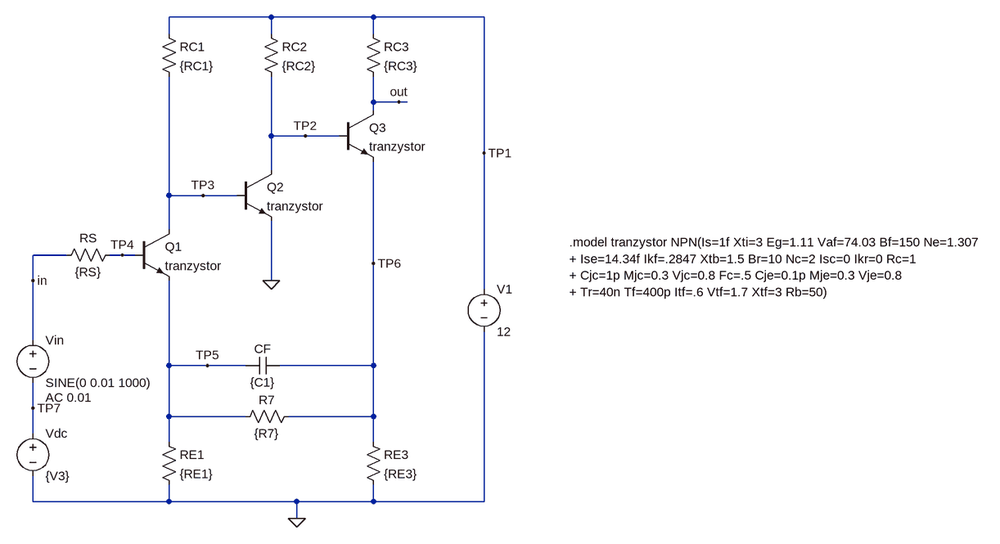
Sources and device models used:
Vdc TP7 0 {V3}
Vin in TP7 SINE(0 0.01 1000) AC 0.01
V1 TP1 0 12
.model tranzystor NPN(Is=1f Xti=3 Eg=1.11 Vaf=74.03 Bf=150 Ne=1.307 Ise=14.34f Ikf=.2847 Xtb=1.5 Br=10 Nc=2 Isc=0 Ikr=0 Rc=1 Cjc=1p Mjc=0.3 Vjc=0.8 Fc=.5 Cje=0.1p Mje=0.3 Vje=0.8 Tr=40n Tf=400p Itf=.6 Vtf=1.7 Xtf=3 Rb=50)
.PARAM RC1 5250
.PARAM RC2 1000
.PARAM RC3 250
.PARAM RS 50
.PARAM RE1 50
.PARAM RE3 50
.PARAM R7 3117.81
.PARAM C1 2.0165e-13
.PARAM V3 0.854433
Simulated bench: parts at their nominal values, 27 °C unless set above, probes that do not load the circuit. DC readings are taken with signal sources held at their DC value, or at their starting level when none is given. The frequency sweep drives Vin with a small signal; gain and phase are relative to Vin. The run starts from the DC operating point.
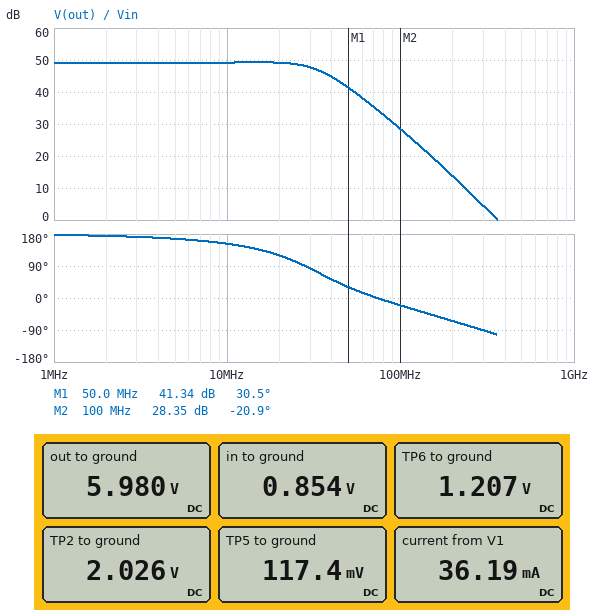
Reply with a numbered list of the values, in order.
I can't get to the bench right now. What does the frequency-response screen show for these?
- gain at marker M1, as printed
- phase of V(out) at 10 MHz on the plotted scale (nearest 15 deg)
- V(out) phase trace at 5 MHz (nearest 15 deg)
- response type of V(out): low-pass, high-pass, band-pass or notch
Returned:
1. 41.34 dB
2. 150 deg
3. 165 deg
4. low-pass
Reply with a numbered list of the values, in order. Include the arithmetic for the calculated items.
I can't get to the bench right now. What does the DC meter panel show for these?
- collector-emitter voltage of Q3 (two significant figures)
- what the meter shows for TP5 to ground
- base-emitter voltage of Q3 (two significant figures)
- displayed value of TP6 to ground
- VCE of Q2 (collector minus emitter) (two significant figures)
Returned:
1. 5.98 V - 1.207 V = 4.8 V
2. 117.4 mV
3. 2.026 V - 1.207 V = 820 mV
4. 1.207 V
5. 2.026 V = 2.0 V
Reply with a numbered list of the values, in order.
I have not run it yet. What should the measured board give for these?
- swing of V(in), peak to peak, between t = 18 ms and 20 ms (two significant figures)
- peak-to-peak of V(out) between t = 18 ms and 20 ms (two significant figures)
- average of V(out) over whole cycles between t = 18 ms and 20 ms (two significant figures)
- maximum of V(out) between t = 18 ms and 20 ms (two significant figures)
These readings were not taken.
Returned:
1. 20 mV
2. 5.7 V
3. 6.0 V
4. 8.8 V
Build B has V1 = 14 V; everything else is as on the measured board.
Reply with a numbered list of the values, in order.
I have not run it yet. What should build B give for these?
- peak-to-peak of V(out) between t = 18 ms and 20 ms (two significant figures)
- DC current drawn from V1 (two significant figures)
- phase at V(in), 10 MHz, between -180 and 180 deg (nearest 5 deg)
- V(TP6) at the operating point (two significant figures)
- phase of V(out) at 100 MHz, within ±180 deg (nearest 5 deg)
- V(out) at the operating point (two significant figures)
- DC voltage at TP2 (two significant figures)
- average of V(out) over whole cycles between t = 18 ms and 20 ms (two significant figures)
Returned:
1. 2.5 V
2. 16 mA
3. 0 deg
4. 1.8 mV
5. -65 deg
6. 14 V
7. 160 mV
8. 13 V
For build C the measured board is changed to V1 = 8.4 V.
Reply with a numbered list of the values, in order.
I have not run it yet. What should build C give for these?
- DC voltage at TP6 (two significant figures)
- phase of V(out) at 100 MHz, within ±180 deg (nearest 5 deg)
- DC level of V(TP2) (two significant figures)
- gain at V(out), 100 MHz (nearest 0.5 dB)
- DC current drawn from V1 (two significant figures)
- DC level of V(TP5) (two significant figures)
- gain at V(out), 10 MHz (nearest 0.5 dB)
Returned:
1. 1.6 V
2. 60 deg
3. 2.7 V
4. -41.5 dB
5. 34 mA
6. 110 mV
7. -48.5 dB
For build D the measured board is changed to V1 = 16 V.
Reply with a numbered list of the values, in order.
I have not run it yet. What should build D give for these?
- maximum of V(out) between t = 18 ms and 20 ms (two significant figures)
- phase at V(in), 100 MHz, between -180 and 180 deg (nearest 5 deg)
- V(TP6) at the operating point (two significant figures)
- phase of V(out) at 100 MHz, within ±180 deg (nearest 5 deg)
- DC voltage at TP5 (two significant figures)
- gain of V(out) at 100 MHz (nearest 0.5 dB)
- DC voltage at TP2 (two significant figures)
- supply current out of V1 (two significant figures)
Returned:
1. 16 V
2. 0 deg
3. 1.8 mV
4. -135 deg
5. 110 mV
6. -59.0 dB
7. 66 mV
8. 19 mA
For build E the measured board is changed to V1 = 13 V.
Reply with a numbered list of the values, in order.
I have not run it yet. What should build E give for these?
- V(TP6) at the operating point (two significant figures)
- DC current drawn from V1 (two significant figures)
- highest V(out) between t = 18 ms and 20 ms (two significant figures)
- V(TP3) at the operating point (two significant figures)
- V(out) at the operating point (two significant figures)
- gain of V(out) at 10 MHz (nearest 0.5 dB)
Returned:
1. 570 mV
2. 25 mA
3. 13 V
4. 790 mV
5. 10 V
6. 49.0 dB
